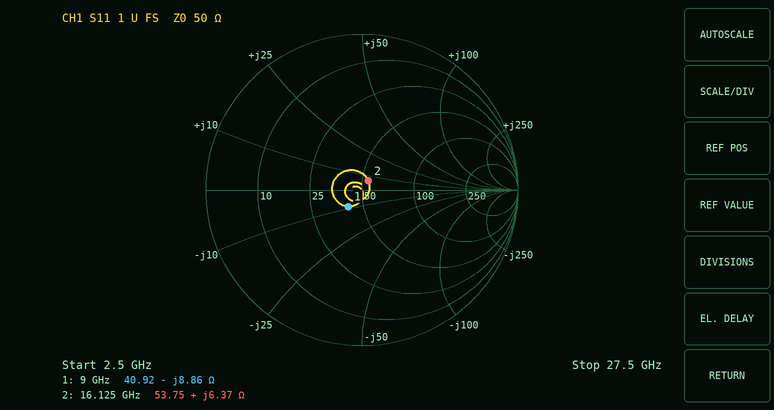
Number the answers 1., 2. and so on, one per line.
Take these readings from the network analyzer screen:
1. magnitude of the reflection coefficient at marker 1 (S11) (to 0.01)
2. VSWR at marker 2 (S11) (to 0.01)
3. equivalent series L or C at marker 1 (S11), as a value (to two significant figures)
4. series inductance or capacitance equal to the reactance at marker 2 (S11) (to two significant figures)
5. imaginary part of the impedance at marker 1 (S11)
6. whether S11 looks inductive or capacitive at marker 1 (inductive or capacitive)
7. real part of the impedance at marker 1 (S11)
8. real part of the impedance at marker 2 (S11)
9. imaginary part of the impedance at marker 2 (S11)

1. 0.14
2. 1.15
3. 2.0 pF
4. 63 pH
5. -8.86 Ω
6. capacitive
7. 40.92 Ω
8. 53.75 Ω
9. +6.37 Ω
